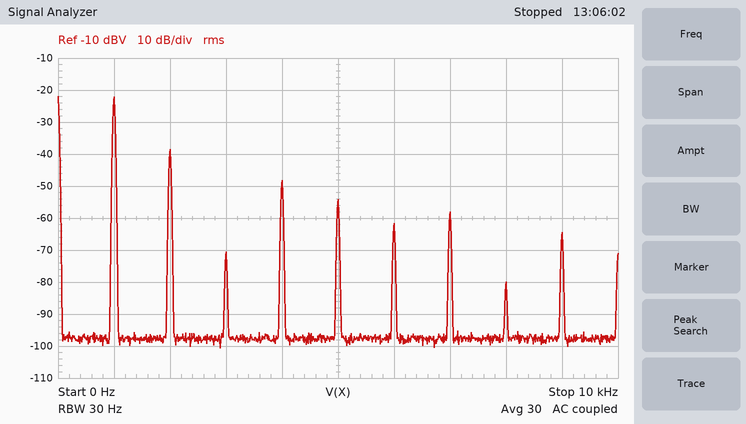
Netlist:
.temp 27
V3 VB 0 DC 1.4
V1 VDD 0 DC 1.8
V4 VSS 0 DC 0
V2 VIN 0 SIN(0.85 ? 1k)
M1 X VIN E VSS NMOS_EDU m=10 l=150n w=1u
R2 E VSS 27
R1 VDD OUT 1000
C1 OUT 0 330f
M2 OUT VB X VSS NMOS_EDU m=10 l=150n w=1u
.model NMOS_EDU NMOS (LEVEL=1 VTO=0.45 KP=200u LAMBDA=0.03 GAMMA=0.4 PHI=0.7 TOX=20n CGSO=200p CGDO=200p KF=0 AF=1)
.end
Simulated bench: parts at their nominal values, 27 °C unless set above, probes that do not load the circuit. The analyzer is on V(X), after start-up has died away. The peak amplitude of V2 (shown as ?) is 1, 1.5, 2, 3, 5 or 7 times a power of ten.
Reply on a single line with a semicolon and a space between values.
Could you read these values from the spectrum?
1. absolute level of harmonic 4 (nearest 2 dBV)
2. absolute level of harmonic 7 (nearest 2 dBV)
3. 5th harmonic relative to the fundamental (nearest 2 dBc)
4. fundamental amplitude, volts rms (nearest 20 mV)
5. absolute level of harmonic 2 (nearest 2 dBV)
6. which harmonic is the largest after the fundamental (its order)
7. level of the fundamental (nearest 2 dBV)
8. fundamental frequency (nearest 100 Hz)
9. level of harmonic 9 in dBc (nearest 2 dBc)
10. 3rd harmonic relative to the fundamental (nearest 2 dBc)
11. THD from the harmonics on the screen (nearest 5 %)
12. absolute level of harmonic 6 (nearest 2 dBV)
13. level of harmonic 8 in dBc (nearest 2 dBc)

-48 dBV; -58 dBV; -32 dBc; 80 mV; -38 dBV; 2; -22 dBV; 1.0 kHz; -42 dBc; -48 dBc; 15 %; -62 dBV; -58 dBc
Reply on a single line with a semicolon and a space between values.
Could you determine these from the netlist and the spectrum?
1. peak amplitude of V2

100 mV
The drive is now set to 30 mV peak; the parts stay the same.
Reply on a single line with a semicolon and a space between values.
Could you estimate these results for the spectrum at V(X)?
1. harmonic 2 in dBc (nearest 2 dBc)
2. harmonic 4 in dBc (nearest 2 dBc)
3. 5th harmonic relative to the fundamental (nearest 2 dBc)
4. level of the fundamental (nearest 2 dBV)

-18 dBc; -38 dBc; -46 dBc; -34 dBV
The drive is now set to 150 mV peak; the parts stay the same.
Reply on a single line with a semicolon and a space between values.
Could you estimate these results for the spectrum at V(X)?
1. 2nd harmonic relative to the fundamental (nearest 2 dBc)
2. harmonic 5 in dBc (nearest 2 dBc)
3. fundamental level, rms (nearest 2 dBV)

-20 dBc; -42 dBc; -20 dBV
